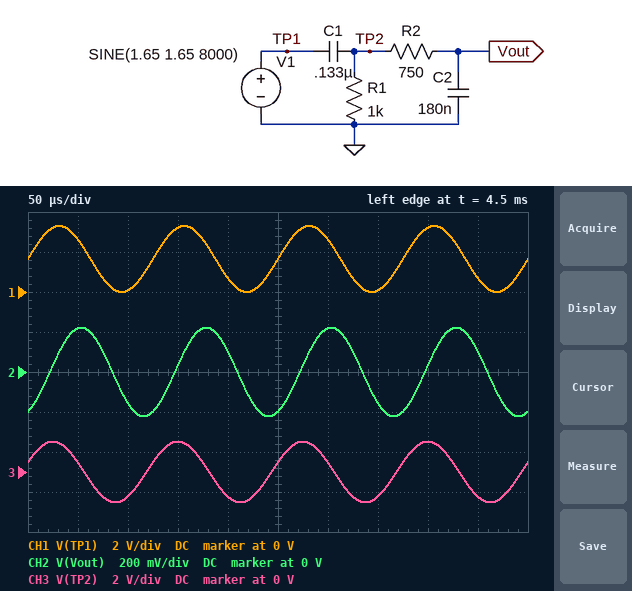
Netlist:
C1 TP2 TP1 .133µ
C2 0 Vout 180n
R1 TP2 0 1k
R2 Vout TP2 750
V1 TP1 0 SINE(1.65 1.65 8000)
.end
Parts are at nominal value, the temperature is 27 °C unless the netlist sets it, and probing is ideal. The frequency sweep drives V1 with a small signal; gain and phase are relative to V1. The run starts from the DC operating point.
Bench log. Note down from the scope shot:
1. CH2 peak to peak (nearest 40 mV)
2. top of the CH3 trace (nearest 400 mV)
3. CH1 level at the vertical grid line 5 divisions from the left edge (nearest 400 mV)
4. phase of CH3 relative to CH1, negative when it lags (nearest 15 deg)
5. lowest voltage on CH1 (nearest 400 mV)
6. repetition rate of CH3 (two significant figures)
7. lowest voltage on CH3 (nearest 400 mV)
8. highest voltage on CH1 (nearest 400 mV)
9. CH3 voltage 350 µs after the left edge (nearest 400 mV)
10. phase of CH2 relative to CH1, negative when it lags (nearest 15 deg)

440 mV
1.6 V
1.6 V
15 deg
0 V
8.0 kHz
-1.6 V
3.2 V
-1.2 V
-60 deg
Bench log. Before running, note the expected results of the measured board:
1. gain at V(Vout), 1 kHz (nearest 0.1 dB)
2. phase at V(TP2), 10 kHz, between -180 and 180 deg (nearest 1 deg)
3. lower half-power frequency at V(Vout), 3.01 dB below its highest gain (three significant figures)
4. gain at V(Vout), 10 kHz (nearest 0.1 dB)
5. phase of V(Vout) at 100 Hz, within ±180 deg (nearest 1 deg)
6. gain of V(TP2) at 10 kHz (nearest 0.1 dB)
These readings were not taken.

-10.6 dB
15 deg
328 Hz
-19.1 dB
74 deg
-0.5 dB
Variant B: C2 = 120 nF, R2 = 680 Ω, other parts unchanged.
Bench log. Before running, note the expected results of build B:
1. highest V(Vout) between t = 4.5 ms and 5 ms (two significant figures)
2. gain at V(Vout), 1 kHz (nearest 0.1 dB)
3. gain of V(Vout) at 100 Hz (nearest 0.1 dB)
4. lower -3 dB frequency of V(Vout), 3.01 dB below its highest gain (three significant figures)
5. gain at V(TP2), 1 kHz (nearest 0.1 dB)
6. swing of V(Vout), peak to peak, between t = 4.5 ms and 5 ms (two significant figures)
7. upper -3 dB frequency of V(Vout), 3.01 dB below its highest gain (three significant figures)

350 mV
-8.3 dB
-21.7 dB
437 Hz
-7.3 dB
700 mV
5.34 kHz
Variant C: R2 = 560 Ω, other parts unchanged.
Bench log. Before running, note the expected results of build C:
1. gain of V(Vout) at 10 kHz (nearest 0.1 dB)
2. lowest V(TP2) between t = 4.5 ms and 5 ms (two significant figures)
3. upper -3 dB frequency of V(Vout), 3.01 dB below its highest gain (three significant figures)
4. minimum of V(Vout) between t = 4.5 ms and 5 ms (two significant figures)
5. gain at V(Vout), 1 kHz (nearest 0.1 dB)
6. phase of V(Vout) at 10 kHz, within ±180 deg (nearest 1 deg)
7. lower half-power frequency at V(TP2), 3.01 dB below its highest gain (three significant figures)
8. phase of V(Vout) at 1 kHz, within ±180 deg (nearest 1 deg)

-16.8 dB
-1.5 V
5.27 kHz
-280 mV
-10.0 dB
-63 deg
3.95 kHz
10 deg
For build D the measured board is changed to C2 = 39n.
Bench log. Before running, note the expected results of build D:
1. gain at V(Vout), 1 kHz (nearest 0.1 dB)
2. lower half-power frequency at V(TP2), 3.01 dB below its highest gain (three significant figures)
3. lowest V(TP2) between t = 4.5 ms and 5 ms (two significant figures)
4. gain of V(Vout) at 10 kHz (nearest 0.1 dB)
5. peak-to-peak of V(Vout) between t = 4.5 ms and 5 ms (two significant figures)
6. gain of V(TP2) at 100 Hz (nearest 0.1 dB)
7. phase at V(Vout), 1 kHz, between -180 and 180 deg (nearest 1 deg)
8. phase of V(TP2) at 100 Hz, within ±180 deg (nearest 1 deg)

-5.2 dB
2.16 kHz
-1.5 V
-7.2 dB
1.6 V
-21.6 dB
34 deg
84 deg
